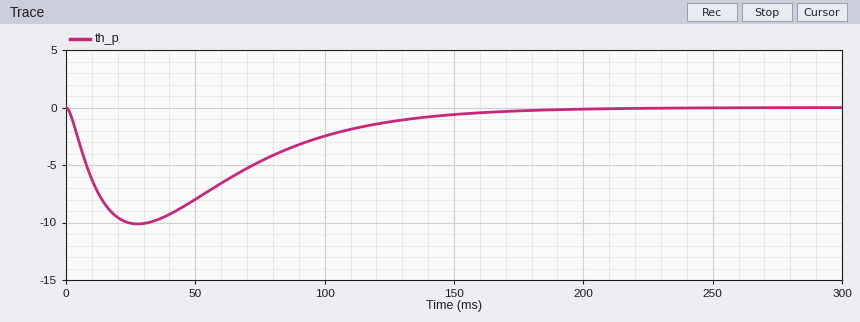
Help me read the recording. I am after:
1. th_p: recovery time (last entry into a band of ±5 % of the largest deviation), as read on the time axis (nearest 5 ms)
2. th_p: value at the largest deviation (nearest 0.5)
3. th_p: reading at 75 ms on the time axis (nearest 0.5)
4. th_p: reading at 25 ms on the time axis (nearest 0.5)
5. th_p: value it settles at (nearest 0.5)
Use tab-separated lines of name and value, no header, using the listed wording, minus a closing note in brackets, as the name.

th_p: recovery time (last entry into a band of ±5 % of the largest deviation), as read on the time axis	155 ms
th_p: value at the largest deviation	-10.0
th_p: reading at 75 ms on the time axis	-4.5
th_p: reading at 25 ms on the time axis	-10.0
th_p: value it settles at	0.0
